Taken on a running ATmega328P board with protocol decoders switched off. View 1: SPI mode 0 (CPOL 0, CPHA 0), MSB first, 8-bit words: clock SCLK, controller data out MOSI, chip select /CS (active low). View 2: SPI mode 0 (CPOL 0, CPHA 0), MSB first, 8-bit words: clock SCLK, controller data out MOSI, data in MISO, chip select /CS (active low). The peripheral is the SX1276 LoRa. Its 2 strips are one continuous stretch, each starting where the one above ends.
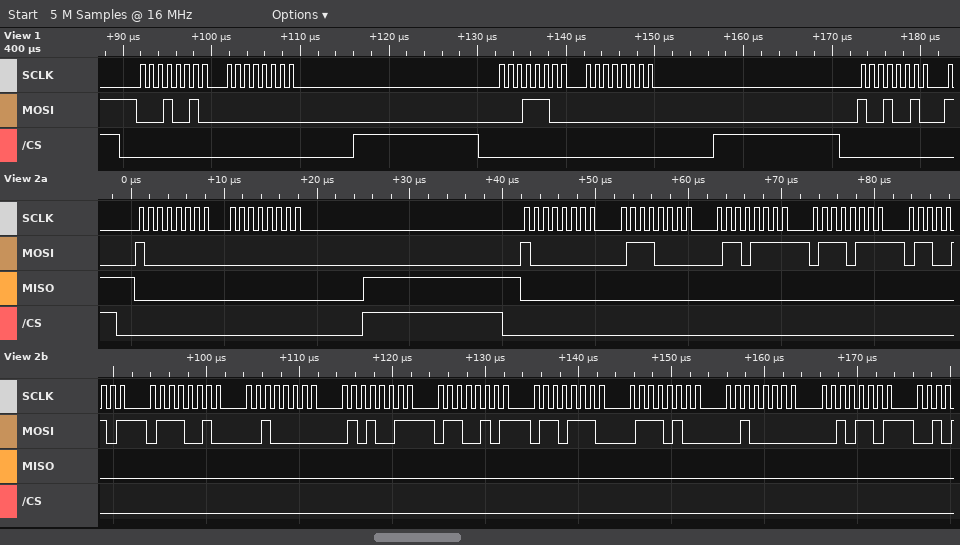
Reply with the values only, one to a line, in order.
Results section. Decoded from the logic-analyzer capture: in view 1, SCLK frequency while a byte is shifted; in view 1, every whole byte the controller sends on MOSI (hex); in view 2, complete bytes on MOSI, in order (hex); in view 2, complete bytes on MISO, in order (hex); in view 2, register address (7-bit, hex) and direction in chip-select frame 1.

1 MHz
0x12 0x00 0x1C 0x00 0x92
80 00 80 70 6F 77 65 72 20 53 65 6E 74 20 2D
00 00 00 00 00 00 00 00 00 00 00 00 00 00 00
0x00 write
